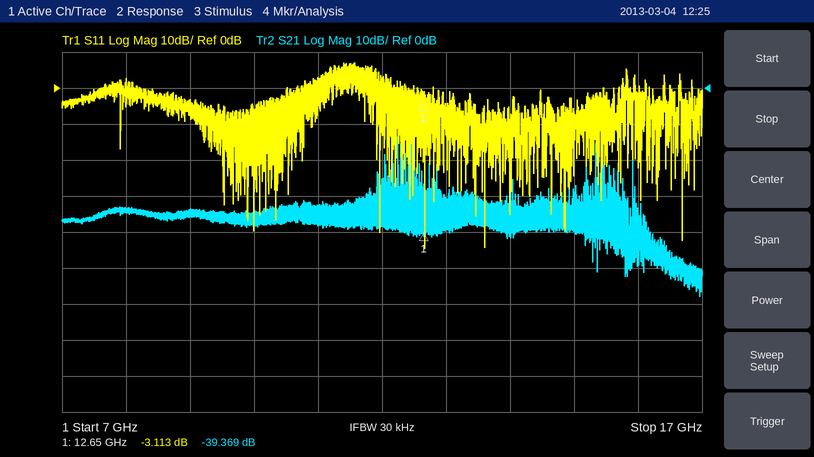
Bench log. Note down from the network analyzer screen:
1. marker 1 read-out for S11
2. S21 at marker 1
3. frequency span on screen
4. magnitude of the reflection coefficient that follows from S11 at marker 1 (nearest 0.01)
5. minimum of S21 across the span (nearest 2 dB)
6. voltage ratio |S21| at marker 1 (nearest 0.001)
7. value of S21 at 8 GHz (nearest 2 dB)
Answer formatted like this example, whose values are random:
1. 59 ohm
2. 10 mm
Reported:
1. -3.113 dB
2. -39.369 dB
3. 10 GHz
4. 0.70
5. -58 dB
6. 0.011
7. -34 dB
